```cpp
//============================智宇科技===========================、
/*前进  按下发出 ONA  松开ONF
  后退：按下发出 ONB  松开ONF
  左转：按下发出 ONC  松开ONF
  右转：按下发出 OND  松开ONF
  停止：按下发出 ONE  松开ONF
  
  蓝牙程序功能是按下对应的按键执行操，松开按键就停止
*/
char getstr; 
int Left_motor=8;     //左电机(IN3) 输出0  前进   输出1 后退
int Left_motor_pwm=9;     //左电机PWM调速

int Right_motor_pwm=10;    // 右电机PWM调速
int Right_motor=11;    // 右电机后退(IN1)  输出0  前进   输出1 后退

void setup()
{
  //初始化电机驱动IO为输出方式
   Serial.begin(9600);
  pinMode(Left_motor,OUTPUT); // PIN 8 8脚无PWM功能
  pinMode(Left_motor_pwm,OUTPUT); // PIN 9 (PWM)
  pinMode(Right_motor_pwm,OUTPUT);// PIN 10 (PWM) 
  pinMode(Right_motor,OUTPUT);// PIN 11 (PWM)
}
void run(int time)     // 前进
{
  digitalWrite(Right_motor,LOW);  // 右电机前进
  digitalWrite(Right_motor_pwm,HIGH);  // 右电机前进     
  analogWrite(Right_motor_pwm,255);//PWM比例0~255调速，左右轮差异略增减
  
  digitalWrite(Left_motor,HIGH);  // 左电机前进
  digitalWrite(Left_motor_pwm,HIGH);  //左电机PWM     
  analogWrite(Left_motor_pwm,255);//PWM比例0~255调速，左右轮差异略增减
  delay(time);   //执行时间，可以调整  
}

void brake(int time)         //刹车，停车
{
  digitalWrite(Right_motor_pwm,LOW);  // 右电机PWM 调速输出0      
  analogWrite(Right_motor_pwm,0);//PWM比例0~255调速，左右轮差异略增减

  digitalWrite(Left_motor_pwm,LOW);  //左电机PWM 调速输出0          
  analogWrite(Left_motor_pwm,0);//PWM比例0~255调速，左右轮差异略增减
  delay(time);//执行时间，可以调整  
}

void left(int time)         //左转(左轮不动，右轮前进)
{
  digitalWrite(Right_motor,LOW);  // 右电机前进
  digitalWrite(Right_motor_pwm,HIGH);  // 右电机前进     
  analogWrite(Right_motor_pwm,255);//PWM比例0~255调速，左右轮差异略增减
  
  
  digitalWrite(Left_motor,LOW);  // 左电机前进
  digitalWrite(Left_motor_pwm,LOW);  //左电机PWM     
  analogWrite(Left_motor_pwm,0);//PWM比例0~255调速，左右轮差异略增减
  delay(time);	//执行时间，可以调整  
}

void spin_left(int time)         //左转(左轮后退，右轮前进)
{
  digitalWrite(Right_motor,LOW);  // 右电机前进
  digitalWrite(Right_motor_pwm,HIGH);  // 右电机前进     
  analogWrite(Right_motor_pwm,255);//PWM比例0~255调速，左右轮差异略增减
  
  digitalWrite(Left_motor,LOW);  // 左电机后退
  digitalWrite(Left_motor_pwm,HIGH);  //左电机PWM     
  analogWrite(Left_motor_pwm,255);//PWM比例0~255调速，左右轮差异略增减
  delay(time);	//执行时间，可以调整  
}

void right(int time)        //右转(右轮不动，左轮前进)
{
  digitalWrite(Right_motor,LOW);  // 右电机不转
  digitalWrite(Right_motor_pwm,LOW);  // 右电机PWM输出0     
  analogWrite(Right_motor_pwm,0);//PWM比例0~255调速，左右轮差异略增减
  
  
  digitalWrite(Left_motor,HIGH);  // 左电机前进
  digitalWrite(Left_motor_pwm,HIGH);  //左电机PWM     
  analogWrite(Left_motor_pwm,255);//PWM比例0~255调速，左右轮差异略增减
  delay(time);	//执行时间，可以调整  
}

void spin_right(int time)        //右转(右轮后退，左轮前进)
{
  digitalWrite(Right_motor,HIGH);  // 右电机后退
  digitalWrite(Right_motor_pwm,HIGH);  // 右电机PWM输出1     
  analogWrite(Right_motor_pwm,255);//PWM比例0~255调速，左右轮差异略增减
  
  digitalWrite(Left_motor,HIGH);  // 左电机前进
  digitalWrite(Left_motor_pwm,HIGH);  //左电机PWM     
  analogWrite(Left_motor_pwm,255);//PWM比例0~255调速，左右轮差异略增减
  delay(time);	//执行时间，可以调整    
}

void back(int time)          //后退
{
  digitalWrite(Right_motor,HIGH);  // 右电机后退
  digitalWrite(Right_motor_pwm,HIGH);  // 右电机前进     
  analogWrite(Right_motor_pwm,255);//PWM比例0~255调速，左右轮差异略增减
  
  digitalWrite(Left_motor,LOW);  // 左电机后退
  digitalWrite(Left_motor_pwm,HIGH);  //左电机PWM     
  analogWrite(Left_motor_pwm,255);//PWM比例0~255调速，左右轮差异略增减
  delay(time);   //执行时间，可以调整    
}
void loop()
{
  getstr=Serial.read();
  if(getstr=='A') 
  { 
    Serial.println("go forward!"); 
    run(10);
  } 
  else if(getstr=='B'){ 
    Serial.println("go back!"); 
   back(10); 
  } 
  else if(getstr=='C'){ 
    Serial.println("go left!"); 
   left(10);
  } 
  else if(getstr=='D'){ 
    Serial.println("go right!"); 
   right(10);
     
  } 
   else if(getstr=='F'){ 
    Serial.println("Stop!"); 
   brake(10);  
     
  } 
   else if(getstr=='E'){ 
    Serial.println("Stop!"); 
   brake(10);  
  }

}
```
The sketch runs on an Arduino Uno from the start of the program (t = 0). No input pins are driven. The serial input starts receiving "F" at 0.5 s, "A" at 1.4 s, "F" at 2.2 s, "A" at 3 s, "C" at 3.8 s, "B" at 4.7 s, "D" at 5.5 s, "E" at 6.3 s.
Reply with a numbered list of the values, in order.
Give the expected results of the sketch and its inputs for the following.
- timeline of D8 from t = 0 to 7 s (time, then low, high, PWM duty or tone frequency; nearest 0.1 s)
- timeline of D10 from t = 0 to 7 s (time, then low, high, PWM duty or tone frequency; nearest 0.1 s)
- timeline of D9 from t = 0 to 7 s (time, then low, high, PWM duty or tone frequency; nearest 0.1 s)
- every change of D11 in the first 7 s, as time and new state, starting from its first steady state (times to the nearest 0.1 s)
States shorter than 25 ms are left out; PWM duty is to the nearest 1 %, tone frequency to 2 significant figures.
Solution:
1. 0 s low; 1.4 s high; 3.8 s low; 5.5 s high
2. 0 s low; 1.4 s high; 2.2 s low; 3 s high; 5.5 s low
3. 0 s low; 1.4 s high; 2.2 s low; 3 s high; 3.8 s low; 4.7 s high; 6.3 s low
4. 0 s low; 4.7 s high; 5.5 s low
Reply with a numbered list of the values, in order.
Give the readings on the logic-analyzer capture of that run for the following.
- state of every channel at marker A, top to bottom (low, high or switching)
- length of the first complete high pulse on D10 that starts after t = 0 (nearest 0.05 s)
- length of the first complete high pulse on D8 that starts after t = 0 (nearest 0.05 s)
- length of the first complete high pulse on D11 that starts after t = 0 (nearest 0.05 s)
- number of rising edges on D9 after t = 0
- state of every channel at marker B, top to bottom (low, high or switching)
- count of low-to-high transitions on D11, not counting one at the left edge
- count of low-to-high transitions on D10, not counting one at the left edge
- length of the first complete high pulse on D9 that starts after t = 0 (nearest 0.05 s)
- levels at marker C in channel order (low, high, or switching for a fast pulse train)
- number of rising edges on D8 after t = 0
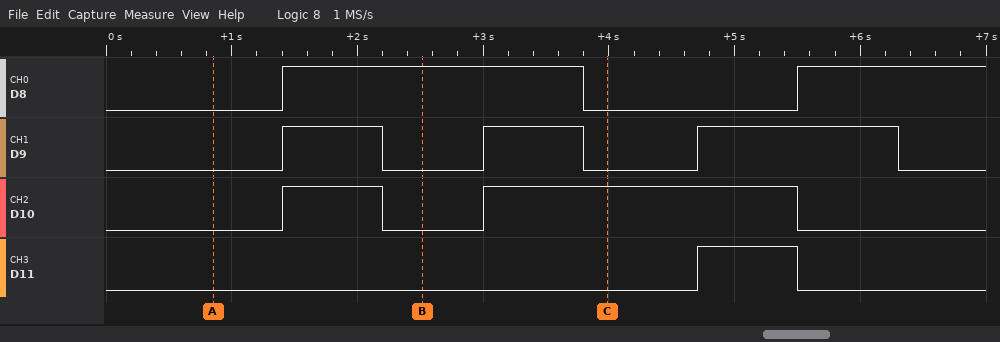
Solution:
1. D8 low, D9 low, D10 low, D11 low
2. 0.80 s
3. 2.40 s
4. 0.80 s
5. 3
6. D8 high, D9 low, D10 low, D11 low
7. 1
8. 2
9. 0.80 s
10. D8 low, D9 low, D10 high, D11 low
11. 2
